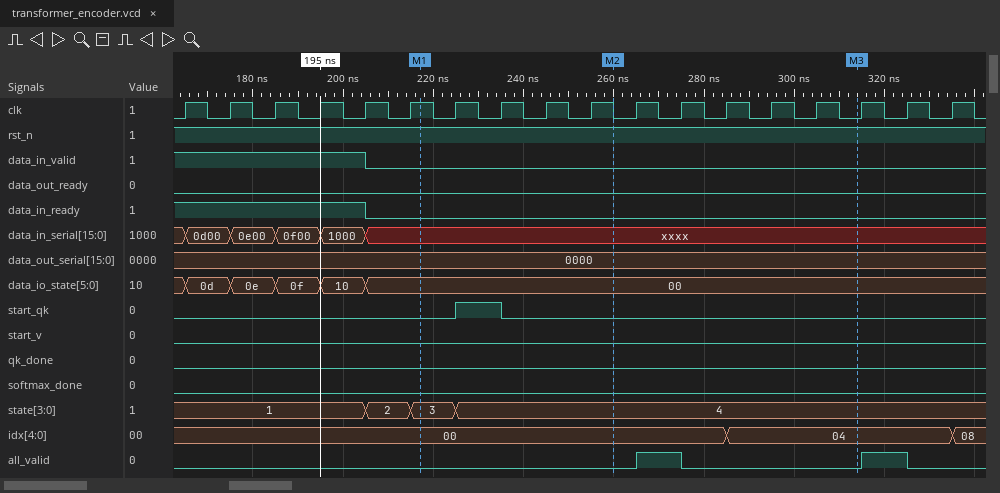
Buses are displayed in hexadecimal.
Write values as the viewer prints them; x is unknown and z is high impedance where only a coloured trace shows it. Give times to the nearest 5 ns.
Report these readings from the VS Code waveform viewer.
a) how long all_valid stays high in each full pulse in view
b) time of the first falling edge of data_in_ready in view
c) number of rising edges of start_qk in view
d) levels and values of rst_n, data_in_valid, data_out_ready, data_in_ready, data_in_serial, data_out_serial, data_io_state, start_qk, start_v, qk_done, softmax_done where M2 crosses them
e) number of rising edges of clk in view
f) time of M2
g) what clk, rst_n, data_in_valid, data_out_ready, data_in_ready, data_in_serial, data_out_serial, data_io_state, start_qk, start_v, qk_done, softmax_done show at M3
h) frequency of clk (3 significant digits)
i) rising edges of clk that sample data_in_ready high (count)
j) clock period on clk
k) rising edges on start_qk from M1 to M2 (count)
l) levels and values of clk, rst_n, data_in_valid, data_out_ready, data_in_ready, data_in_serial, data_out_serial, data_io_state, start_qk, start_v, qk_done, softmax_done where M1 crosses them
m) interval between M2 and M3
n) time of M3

10 ns, 10 ns
205 ns
1
rst_n=1, data_in_valid=0, data_out_ready=0, data_in_ready=0, data_in_serial=xxxx, data_out_serial=0000, data_io_state=00, start_qk=0, start_v=0, qk_done=0, softmax_done=0
18
260 ns
clk=0, rst_n=1, data_in_valid=0, data_out_ready=0, data_in_ready=0, data_in_serial=xxxx, data_out_serial=0000, data_io_state=00, start_qk=0, start_v=0, qk_done=0, softmax_done=0
100 MHz
5
10 ns
1
clk=1, rst_n=1, data_in_valid=0, data_out_ready=0, data_in_ready=0, data_in_serial=xxxx, data_out_serial=0000, data_io_state=00, start_qk=0, start_v=0, qk_done=0, softmax_done=0
55 ns
315 ns
